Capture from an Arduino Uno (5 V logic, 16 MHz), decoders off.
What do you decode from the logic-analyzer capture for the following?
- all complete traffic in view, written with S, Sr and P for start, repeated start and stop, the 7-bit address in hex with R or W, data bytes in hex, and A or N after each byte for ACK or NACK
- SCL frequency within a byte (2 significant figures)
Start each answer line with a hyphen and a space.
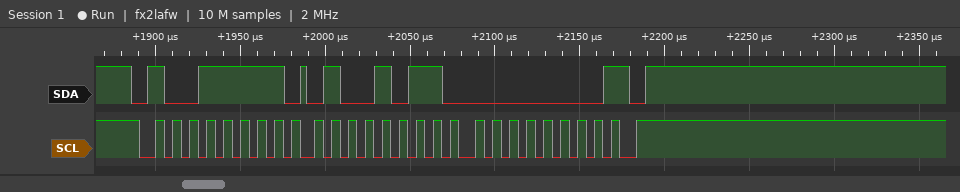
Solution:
- S 4FR A 4B A 00 N P
- 100 kHz
